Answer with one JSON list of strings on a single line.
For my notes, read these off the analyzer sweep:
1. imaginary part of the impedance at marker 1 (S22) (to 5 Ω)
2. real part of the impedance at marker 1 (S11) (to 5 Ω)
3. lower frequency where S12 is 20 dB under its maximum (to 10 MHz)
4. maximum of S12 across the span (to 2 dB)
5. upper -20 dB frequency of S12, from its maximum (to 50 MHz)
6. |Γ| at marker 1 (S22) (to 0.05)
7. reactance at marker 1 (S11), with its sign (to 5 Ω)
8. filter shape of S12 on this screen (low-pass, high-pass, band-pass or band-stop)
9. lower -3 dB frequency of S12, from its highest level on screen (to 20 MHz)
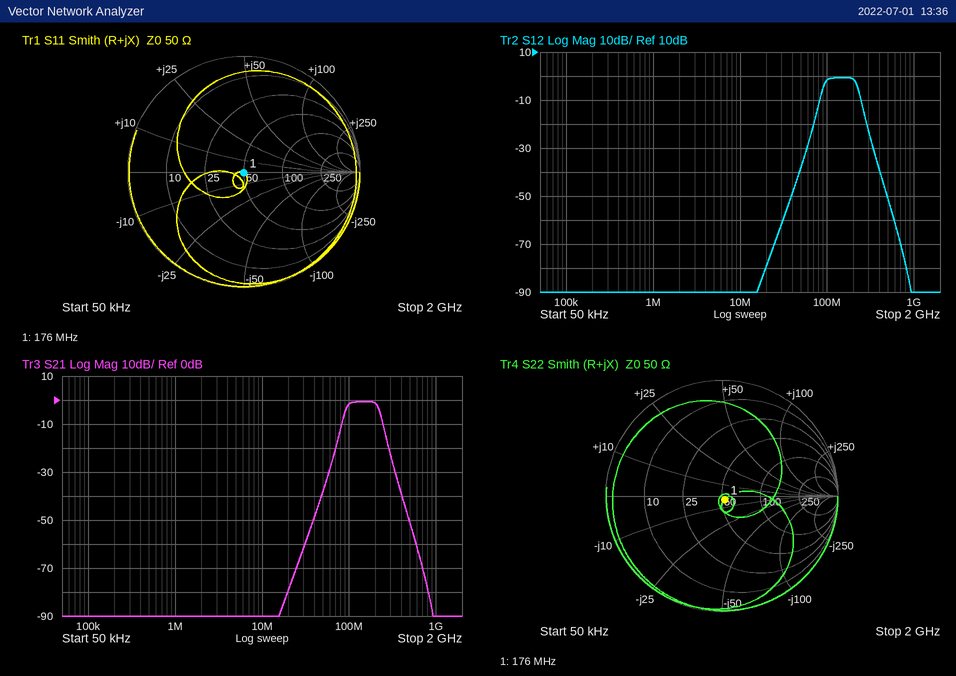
["-5 Ω", "50 Ω", "70 MHz", "0 dB", "300 MHz", "0.05", "0 Ω", "band-pass", "100 MHz"]
